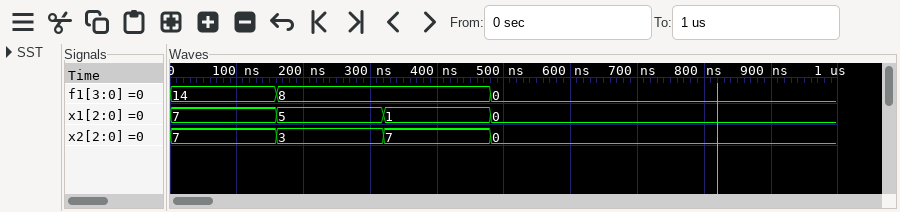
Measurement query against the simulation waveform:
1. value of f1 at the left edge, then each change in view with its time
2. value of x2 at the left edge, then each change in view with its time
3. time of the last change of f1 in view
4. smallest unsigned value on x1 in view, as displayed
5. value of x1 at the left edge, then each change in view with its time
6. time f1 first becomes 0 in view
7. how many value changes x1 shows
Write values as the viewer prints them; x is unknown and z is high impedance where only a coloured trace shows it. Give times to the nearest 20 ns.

14, 8 at 160 ns, 0 at 480 ns
7, 3 at 160 ns, 7 at 320 ns, 0 at 480 ns
480 ns
0
7, 5 at 160 ns, 1 at 320 ns, 0 at 480 ns
480 ns
3
